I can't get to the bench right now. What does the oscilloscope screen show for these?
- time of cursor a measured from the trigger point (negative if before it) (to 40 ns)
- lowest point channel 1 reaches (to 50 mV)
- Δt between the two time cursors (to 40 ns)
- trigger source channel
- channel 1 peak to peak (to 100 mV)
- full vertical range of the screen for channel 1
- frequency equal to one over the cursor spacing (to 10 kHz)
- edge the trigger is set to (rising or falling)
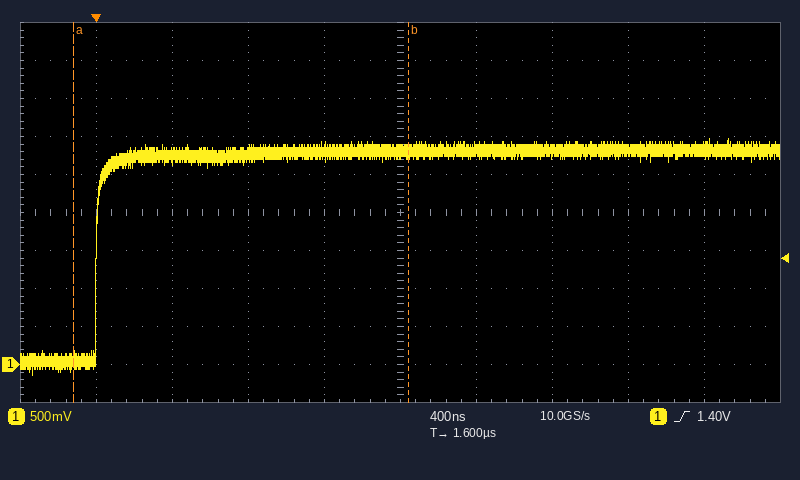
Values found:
-120 ns
-150 mV
1.76 µs
channel 1
3.10 V
5 V
570 kHz
rising
